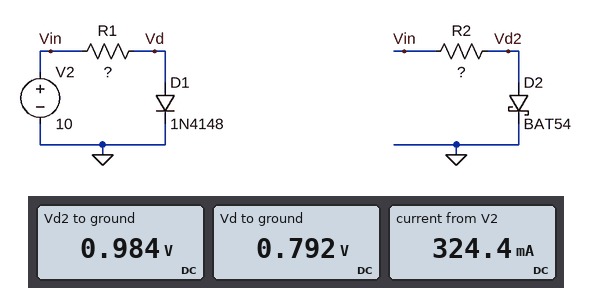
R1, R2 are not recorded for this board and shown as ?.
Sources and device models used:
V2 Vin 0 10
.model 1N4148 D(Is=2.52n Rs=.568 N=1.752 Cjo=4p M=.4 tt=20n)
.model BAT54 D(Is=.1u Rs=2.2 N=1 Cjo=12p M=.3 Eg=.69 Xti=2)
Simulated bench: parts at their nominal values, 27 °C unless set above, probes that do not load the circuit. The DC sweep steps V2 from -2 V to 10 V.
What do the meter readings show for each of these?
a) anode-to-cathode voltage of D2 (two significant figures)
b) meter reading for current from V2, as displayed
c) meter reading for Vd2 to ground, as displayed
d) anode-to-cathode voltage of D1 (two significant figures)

980 mV
324.4 mA
0.984 V
790 mV
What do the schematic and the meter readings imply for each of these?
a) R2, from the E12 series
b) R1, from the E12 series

33 Ω
180 Ω
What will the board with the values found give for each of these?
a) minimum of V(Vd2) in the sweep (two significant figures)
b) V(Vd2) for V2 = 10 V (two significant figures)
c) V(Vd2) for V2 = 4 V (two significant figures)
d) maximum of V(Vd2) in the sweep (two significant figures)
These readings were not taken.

-2.0 V
980 mV
590 mV
980 mV
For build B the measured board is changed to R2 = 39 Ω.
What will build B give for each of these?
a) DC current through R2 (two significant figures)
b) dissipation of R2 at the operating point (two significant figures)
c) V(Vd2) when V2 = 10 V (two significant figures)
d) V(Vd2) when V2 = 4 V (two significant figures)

230 mA
2.1 W
890 mV
550 mV
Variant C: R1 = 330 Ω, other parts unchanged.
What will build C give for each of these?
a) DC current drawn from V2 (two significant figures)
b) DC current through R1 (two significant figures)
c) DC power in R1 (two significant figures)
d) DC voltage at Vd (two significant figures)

300 mA
28 mA
260 mW
750 mV
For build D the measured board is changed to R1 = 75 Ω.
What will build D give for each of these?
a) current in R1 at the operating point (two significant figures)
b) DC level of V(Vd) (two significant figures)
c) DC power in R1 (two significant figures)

120 mA
870 mV
1.1 W
